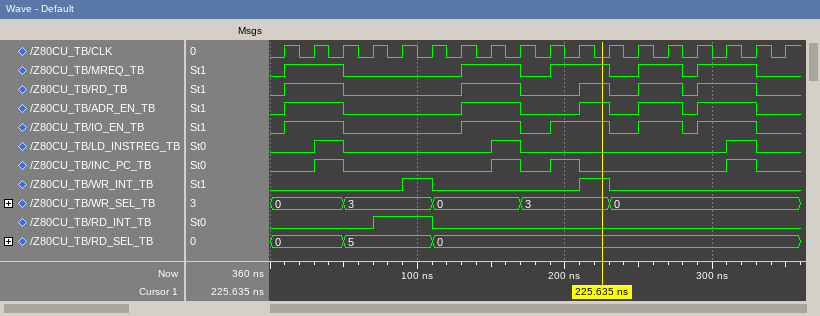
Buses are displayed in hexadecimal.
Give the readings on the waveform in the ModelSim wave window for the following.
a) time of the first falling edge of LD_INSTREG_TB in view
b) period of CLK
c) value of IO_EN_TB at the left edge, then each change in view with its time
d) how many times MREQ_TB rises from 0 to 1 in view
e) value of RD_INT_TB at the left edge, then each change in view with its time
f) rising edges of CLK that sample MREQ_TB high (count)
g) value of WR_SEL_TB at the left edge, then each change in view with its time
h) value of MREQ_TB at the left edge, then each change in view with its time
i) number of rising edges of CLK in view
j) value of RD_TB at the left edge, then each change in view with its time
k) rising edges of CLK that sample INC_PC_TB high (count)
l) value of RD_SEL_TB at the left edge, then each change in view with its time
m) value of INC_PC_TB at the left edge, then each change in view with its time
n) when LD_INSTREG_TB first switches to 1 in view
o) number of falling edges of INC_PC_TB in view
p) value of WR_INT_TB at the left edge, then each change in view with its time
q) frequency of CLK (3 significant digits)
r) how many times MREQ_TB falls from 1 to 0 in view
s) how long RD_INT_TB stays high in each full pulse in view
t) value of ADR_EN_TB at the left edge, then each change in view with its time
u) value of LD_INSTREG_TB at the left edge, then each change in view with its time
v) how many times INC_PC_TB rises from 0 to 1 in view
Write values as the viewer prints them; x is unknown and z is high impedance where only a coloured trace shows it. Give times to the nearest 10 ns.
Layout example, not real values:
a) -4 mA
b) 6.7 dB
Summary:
a) 50 ns
b) 20 ns
c) 0, 1 at 10 ns, 0 at 50 ns, 1 at 130 ns, 0 at 170 ns, 1 at 190 ns, 0 at 230 ns, 1 at 250 ns, 0 at 280 ns, 1 at 290 ns, 0 at 330 ns
d) 5
e) 0, 1 at 70 ns, 0 at 110 ns
f) 9
g) 0, 3 at 50 ns, 0 at 110 ns, 3 at 170 ns, 0 at 230 ns
h) 0, 1 at 10 ns, 0 at 50 ns, 1 at 130 ns, 0 at 170 ns, 1 at 190 ns, 0 at 230 ns, 1 at 250 ns, 0 at 280 ns, 1 at 290 ns, 0 at 330 ns
i) 18
j) 0, 1 at 10 ns, 0 at 50 ns, 1 at 130 ns, 0 at 170 ns, 1 at 210 ns, 0 at 230 ns, 1 at 250 ns, 0 at 280 ns, 1 at 290 ns, 0 at 330 ns
k) 4
l) 0, 5 at 50 ns, 0 at 110 ns
m) 0, 1 at 30 ns, 0 at 50 ns, 1 at 150 ns, 0 at 170 ns, 1 at 190 ns, 0 at 210 ns, 1 at 310 ns, 0 at 330 ns
n) 30 ns
o) 4
p) 0, 1 at 90 ns, 0 at 110 ns, 1 at 210 ns, 0 at 230 ns
q) 50.0 MHz
r) 5
s) 40 ns
t) 0, 1 at 10 ns, 0 at 50 ns, 1 at 130 ns, 0 at 170 ns, 1 at 210 ns, 0 at 230 ns, 1 at 250 ns, 0 at 280 ns, 1 at 290 ns, 0 at 330 ns
u) 0, 1 at 30 ns, 0 at 50 ns, 1 at 150 ns, 0 at 170 ns, 1 at 310 ns, 0 at 330 ns
v) 4
